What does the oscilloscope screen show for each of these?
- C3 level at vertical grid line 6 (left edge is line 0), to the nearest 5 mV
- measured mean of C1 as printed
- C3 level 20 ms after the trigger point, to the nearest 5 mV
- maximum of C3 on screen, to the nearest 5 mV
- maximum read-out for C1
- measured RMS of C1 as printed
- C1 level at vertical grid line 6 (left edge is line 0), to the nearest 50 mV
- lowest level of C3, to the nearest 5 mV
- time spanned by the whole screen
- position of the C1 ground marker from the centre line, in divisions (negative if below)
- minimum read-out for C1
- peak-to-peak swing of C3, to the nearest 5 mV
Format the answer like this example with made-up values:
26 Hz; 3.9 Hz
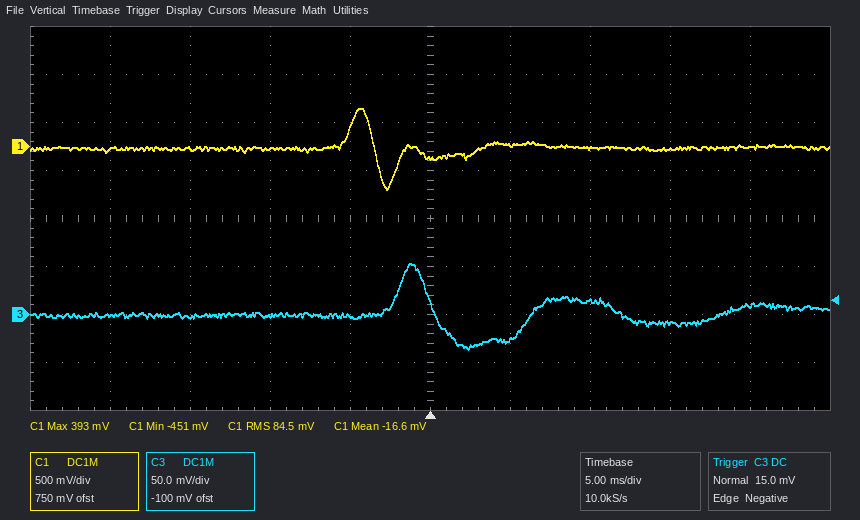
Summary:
-25 mV; -16.6 mV; 10 mV; 55 mV; 393 mV; 84.5 mV; 0 mV; -35 mV; 50 ms; +1.5 div; -451 mV; 90 mV
